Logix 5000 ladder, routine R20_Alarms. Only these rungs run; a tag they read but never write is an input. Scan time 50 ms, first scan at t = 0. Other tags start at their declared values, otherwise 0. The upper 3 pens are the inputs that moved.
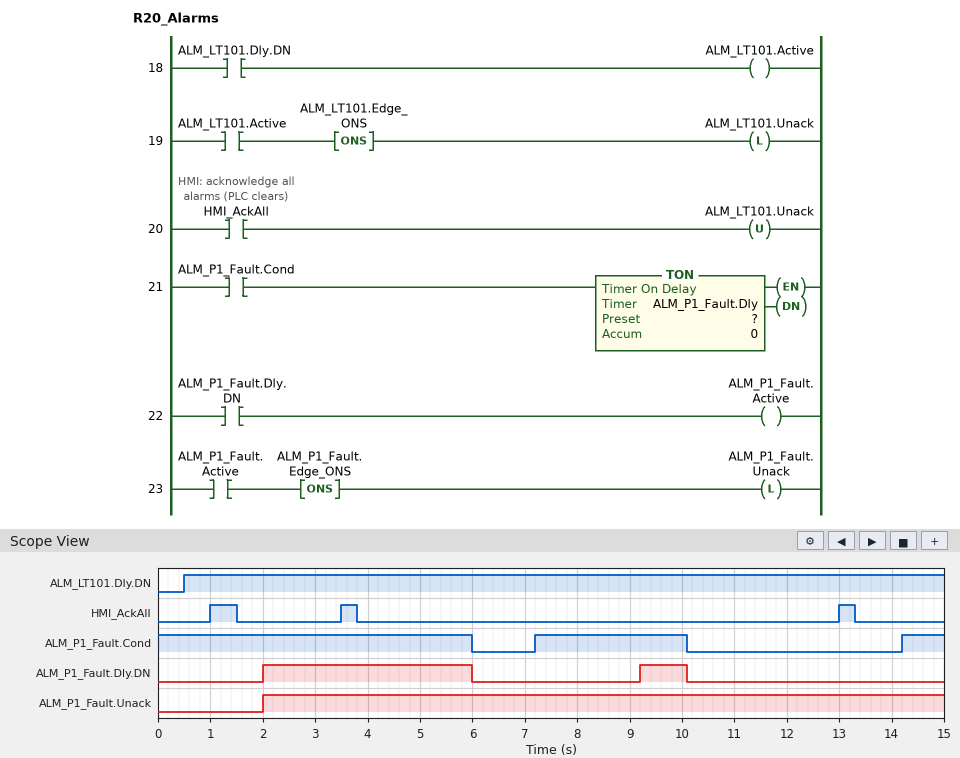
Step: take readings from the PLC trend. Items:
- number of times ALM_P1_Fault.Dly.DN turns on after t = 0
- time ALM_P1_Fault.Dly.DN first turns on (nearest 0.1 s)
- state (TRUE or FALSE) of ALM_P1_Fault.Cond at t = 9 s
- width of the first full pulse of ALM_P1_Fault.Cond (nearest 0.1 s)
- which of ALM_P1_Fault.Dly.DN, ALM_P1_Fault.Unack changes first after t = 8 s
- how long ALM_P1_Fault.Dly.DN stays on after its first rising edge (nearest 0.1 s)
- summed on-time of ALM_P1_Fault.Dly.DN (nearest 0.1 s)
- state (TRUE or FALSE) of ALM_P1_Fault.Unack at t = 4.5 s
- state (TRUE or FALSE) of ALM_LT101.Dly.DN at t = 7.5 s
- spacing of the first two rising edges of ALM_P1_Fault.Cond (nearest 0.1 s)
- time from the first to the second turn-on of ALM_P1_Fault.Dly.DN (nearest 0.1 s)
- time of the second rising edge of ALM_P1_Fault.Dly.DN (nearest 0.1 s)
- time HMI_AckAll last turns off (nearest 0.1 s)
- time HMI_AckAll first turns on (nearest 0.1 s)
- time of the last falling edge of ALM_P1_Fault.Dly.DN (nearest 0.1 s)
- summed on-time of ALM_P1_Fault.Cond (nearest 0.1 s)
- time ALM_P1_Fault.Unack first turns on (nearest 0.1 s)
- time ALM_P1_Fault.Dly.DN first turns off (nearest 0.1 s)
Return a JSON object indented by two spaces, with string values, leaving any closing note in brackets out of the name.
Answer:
{
  "number of times ALM_P1_Fault.Dly.DN turns on after t = 0": "2",
  "time ALM_P1_Fault.Dly.DN first turns on": "2.0 s",
  "state (TRUE or FALSE) of ALM_P1_Fault.Cond at t = 9 s": "TRUE",
  "width of the first full pulse of ALM_P1_Fault.Cond": "2.9 s",
  "which of ALM_P1_Fault.Dly.DN, ALM_P1_Fault.Unack changes first after t = 8 s": "ALM_P1_Fault.Dly.DN",
  "how long ALM_P1_Fault.Dly.DN stays on after its first rising edge": "4.0 s",
  "summed on-time of ALM_P1_Fault.Dly.DN": "4.9 s",
  "state (TRUE or FALSE) of ALM_P1_Fault.Unack at t = 4.5 s": "TRUE",
  "state (TRUE or FALSE) of ALM_LT101.Dly.DN at t = 7.5 s": "TRUE",
  "spacing of the first two rising edges of ALM_P1_Fault.Cond": "7.0 s",
  "time from the first to the second turn-on of ALM_P1_Fault.Dly.DN": "7.2 s",
  "time of the second rising edge of ALM_P1_Fault.Dly.DN": "9.2 s",
  "time HMI_AckAll last turns off": "13.3 s",
  "time HMI_AckAll first turns on": "1.0 s",
  "time of the last falling edge of ALM_P1_Fault.Dly.DN": "10.1 s",
  "summed on-time of ALM_P1_Fault.Cond": "9.7 s",
  "time ALM_P1_Fault.Unack first turns on": "2.0 s",
  "time ALM_P1_Fault.Dly.DN first turns off": "6.0 s"
}
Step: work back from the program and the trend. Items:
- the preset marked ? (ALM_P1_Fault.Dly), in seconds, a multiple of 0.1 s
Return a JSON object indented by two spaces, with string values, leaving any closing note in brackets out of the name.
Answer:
{
  "the preset marked ? (ALM_P1_Fault.Dly), in seconds, a multiple of 0.1 s": "2.0 s"
}
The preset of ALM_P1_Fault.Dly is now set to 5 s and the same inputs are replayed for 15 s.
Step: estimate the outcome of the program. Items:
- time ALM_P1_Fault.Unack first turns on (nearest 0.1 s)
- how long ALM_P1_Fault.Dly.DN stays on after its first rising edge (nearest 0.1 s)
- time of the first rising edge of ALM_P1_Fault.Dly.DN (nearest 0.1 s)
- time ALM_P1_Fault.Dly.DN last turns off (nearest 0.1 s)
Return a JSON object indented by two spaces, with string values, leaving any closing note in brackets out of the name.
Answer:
{
  "time ALM_P1_Fault.Unack first turns on": "5.0 s",
  "how long ALM_P1_Fault.Dly.DN stays on after its first rising edge": "1.0 s",
  "time of the first rising edge of ALM_P1_Fault.Dly.DN": "5.0 s",
  "time ALM_P1_Fault.Dly.DN last turns off": "6.0 s"
}
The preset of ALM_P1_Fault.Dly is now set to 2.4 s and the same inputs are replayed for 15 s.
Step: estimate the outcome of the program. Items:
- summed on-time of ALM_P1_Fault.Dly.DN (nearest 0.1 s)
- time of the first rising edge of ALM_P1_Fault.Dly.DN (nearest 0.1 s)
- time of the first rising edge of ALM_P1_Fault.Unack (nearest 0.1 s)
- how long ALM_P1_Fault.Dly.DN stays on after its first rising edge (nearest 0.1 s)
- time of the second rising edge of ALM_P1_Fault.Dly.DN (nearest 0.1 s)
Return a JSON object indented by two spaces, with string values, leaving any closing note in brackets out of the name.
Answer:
{
  "summed on-time of ALM_P1_Fault.Dly.DN": "4.1 s",
  "time of the first rising edge of ALM_P1_Fault.Dly.DN": "2.4 s",
  "time of the first rising edge of ALM_P1_Fault.Unack": "2.4 s",
  "how long ALM_P1_Fault.Dly.DN stays on after its first rising edge": "3.6 s",
  "time of the second rising edge of ALM_P1_Fault.Dly.DN": "9.6 s"
}
